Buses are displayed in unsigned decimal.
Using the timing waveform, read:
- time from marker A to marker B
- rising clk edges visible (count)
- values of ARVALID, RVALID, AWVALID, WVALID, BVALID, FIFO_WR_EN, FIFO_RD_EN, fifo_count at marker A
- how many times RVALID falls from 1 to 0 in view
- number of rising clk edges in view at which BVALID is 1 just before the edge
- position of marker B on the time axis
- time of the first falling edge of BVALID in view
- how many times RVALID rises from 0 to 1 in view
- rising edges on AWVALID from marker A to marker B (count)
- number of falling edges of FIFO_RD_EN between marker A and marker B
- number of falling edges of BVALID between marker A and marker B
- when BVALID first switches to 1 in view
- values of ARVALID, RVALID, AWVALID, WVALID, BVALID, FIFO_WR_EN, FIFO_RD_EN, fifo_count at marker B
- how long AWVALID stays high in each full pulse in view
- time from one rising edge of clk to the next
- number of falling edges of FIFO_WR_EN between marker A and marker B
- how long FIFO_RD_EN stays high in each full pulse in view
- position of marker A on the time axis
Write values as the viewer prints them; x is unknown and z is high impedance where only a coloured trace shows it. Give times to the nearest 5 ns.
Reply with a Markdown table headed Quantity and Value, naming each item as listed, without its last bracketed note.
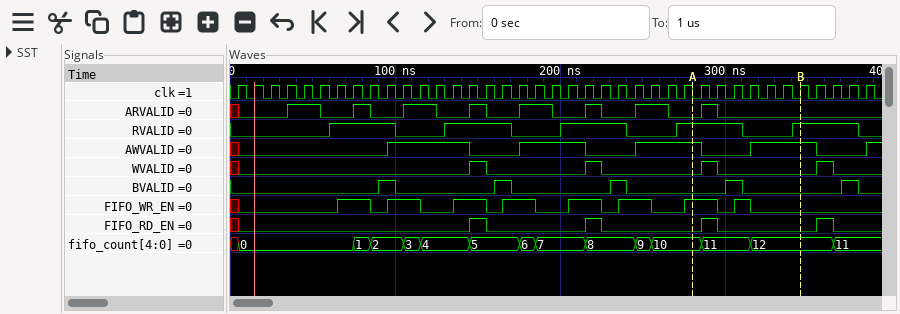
| Quantity | Value |
|---|---|
| time from marker A to marker B | 65 ns |
| rising clk edges visible | 39 |
| values of ARVALID, RVALID, AWVALID, WVALID, BVALID, FIFO_WR_EN, FIFO_RD_EN, fifo_count at marker A | ARVALID=0, RVALID=1, AWVALID=1, WVALID=0, BVALID=0, FIFO_WR_EN=1, FIFO_RD_EN=0, fifo_count=10 |
| how many times RVALID falls from 1 to 0 in view | 5 |
| number of rising clk edges in view at which BVALID is 1 just before the edge | 5 |
| position of marker B on the time axis | 345 ns |
| time of the first falling edge of BVALID in view | 100 ns |
| how many times RVALID rises from 0 to 1 in view | 5 |
| rising edges on AWVALID from marker A to marker B | 1 |
| number of falling edges of FIFO_RD_EN between marker A and marker B | 1 |
| number of falling edges of BVALID between marker A and marker B | 1 |
| when BVALID first switches to 1 in view | 90 ns |
| values of ARVALID, RVALID, AWVALID, WVALID, BVALID, FIFO_WR_EN, FIFO_RD_EN, fifo_count at marker B | ARVALID=0, RVALID=1, AWVALID=1, WVALID=0, BVALID=0, FIFO_WR_EN=0, FIFO_RD_EN=0, fifo_count=12 |
| how long AWVALID stays high in each full pulse in view | 50 ns, 40 ns, 40 ns, 40 ns |
| time from one rising edge of clk to the next | 10 ns |
| number of falling edges of FIFO_WR_EN between marker A and marker B | 2 |
| how long FIFO_RD_EN stays high in each full pulse in view | 10 ns, 10 ns, 10 ns, 10 ns |
| position of marker A on the time axis | 280 ns |
